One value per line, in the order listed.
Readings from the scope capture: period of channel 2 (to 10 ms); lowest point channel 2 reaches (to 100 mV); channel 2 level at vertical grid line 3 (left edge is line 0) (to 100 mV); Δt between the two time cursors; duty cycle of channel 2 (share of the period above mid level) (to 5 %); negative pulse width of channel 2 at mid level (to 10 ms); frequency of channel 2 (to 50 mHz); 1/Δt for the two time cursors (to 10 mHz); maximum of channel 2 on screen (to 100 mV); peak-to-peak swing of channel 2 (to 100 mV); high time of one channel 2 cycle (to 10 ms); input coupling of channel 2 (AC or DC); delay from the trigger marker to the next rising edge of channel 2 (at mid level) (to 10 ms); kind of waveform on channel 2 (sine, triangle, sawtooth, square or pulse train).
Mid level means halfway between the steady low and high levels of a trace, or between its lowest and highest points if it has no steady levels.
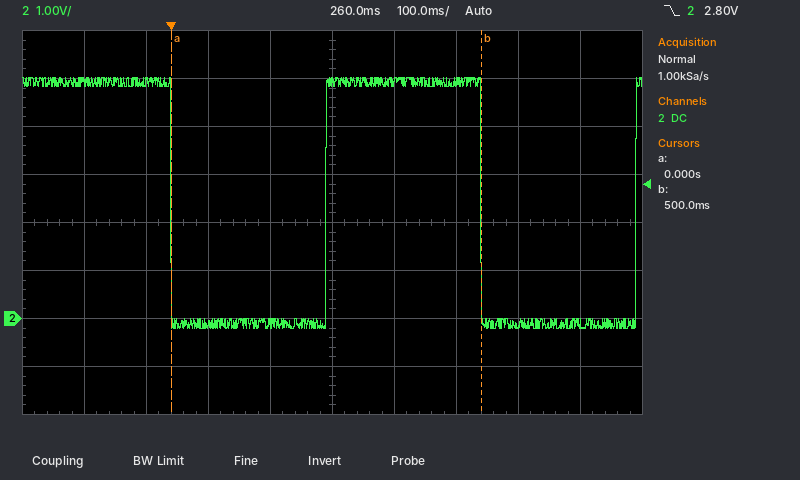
500 ms
-200 mV
-100 mV
500 ms
50 %
250 ms
2.00 Hz
2.00 Hz
5.0 V
5.2 V
250 ms
DC
250 ms
square
